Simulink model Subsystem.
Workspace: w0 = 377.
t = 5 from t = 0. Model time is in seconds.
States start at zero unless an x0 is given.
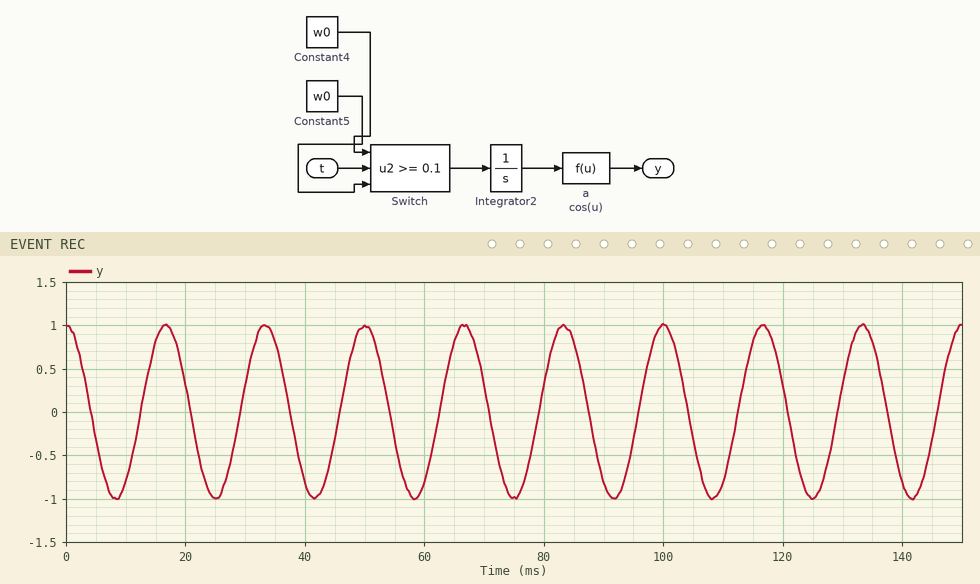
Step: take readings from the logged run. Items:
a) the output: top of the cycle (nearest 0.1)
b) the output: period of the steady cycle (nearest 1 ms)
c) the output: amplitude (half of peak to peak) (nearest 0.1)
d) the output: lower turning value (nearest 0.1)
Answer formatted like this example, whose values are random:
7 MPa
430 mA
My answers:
1.0
17 ms
1.0
-1.0
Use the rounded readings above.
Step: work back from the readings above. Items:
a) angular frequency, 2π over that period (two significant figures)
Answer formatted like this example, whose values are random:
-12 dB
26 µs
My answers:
0.37 rad/ms
